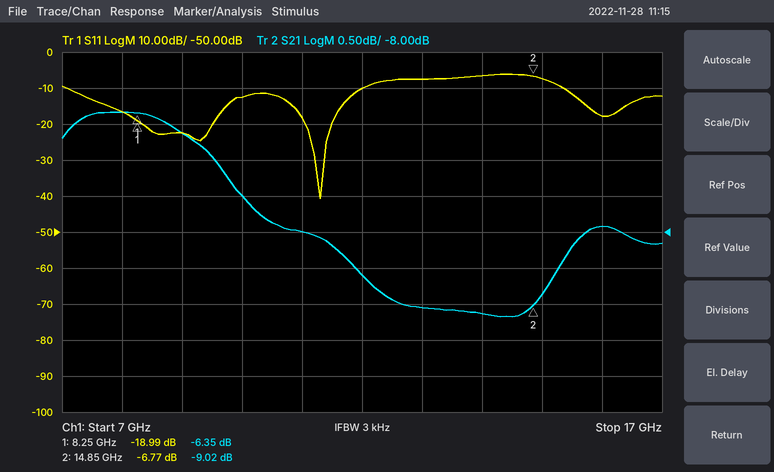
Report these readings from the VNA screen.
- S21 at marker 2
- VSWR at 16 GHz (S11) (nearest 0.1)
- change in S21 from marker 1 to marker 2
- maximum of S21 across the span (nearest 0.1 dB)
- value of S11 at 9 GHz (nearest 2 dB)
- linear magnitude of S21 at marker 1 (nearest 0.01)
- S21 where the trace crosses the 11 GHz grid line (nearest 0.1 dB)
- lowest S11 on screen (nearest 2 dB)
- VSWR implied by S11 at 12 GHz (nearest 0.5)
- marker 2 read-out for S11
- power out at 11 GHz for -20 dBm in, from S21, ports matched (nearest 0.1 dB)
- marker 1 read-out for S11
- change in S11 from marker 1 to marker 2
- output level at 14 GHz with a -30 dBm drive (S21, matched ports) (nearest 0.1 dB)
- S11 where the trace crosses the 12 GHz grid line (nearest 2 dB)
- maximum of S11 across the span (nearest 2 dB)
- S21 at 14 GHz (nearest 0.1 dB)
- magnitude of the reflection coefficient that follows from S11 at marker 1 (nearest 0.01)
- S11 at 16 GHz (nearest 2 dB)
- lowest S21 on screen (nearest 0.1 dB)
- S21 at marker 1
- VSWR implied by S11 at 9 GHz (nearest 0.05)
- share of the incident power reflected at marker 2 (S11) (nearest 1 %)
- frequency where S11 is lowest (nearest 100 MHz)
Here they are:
-9.02 dB
1.3
-2.67 dB
-6.3 dB
-22 dB
0.48
-8.0 dB
-40 dB
2.0
-6.77 dB
-28.0 dBm
-18.99 dB
12.22 dB
-39.1 dBm
-10 dB
-6 dB
-9.1 dB
0.11
-18 dB
-9.2 dB
-6.35 dB
1.15
21 %
11.3 GHz
